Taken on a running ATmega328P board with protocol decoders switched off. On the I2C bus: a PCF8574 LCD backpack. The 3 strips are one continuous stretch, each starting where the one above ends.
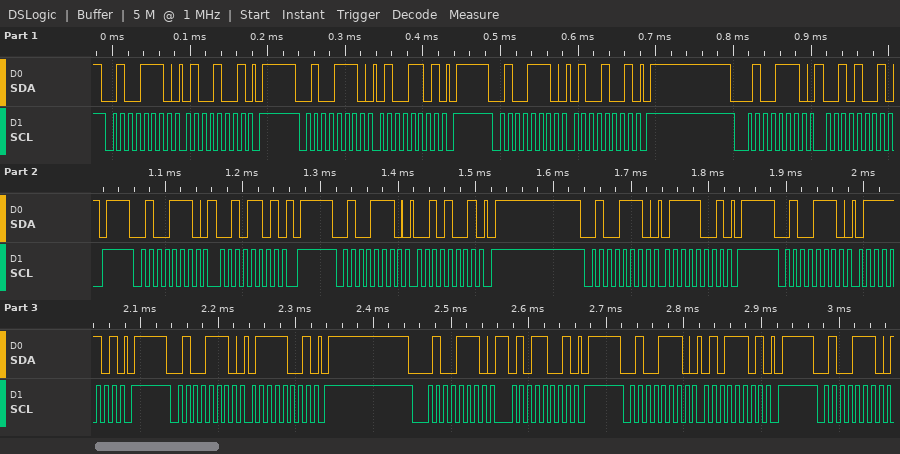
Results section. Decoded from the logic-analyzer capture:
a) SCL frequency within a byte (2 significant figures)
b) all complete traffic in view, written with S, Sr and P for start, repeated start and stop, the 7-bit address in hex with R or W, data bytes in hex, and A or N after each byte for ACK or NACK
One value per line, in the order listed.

100 kHz
S 27W A 49 A P S 27W A 4D A P S 27W A 49 A P S 27W A 29 A P S 27W A 2D A P S 27W A 29 A P S 27W A 79 A P S 27W A 7D A P S 27W A 79 A P S 27W A 59 A P S 27W A 5D A P S 27W A
